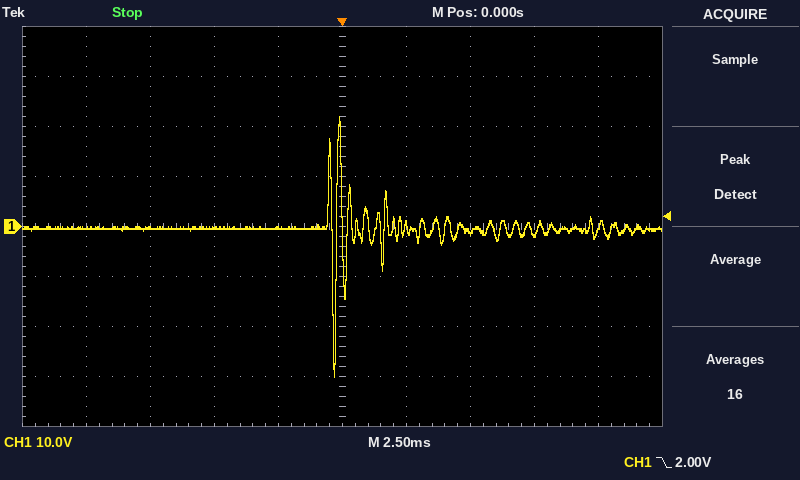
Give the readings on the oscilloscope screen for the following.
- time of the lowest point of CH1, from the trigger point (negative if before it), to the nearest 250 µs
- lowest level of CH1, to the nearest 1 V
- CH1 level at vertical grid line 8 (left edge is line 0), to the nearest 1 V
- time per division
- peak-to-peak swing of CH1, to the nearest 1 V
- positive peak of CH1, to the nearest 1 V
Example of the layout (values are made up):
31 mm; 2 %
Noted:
-250 µs; -30 V; -1 V; 2.5 ms; 52 V; 22 V
